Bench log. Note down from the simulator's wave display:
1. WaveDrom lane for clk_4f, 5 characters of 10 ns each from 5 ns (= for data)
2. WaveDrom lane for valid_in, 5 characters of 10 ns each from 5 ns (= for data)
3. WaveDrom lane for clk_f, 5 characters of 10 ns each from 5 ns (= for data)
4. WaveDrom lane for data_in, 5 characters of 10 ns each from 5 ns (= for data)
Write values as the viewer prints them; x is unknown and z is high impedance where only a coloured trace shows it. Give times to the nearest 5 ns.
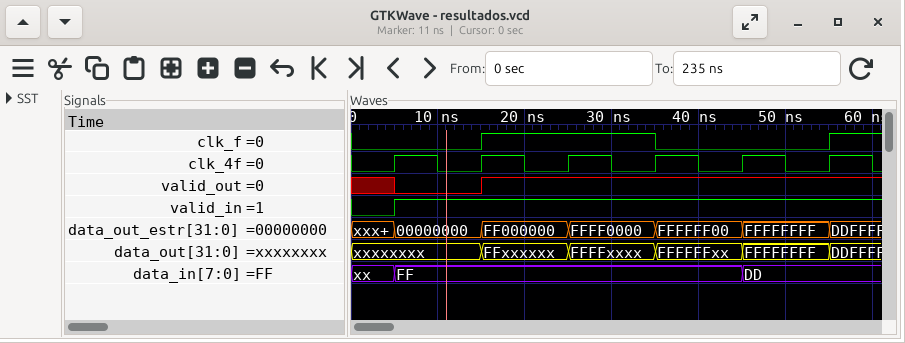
{name: 'clk_4f', wave: 'p....'}
{name: 'valid_in', wave: '1....'}
{name: 'clk_f', wave: '01.0.'}
{name: 'data_in', wave: '=...=', data: 'FF DD'}
